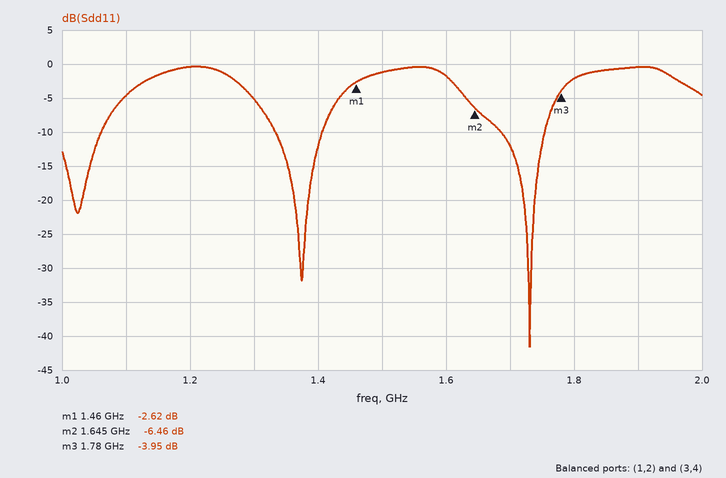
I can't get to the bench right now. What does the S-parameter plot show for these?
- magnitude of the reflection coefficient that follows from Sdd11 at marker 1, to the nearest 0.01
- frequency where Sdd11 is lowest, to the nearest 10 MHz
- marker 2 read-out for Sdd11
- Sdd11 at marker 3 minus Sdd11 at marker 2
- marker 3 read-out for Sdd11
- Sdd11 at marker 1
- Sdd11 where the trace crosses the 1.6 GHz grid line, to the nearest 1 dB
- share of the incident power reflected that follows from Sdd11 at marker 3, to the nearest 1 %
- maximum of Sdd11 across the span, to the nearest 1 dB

0.74
1.73 GHz
-6.46 dB
2.51 dB
-3.95 dB
-2.62 dB
-2 dB
40 %
0 dB
